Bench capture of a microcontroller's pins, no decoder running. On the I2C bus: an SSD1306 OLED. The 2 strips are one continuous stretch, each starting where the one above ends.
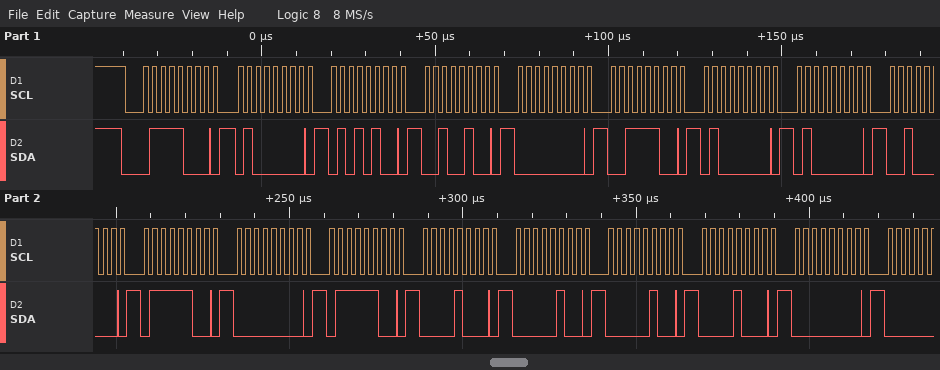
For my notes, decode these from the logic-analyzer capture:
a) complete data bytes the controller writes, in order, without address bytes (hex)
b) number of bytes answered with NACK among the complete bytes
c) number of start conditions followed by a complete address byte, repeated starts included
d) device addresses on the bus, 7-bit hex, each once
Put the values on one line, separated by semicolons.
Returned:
40 54 24 00 3C 40 40 20 7C 00 7C 08 04 04 08 00; 0; 1; 0x3C
